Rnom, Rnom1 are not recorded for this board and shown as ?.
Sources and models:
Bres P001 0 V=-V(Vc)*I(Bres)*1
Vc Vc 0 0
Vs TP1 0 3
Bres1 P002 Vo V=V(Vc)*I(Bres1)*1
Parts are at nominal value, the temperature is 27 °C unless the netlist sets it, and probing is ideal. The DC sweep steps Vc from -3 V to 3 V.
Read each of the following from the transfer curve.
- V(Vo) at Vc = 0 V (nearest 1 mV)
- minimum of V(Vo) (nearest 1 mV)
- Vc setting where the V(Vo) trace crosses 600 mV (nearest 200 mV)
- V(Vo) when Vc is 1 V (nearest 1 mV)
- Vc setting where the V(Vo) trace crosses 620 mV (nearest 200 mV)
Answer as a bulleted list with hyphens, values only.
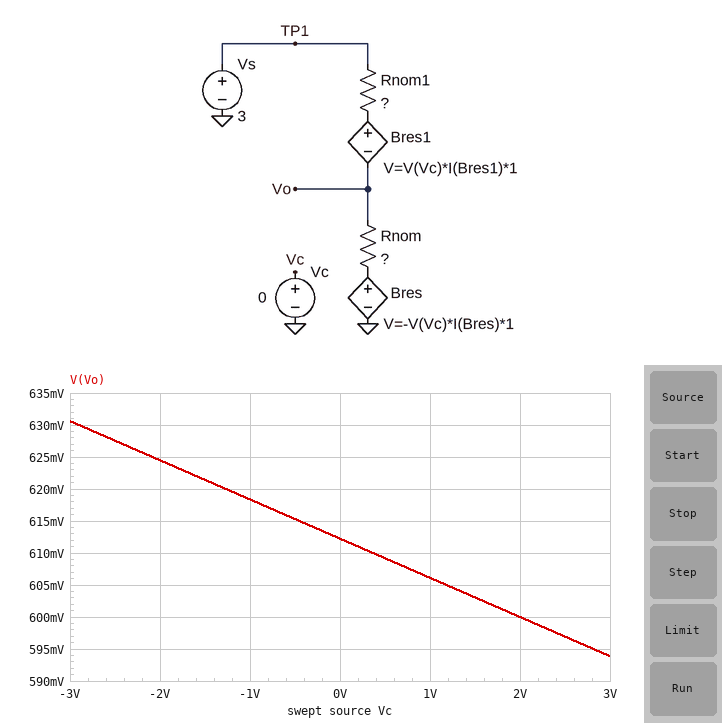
- 612 mV
- 594 mV
- 2.0 V
- 606 mV
- -1.2 V
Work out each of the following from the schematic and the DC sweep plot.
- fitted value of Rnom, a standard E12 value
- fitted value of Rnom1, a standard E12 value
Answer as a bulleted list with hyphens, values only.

- 100 Ω
- 390 Ω
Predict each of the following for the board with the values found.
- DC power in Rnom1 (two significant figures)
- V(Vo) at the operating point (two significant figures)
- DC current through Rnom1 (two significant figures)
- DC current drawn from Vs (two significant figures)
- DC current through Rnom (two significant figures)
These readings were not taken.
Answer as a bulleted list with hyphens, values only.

- 15 mW
- 610 mV
- 6.1 mA
- 6.1 mA
- 6.1 mA
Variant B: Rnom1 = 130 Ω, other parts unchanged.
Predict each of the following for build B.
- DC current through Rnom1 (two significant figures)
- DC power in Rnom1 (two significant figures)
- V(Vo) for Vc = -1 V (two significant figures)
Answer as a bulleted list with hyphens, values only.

- 13 mA
- 22 mW
- 1.3 V
